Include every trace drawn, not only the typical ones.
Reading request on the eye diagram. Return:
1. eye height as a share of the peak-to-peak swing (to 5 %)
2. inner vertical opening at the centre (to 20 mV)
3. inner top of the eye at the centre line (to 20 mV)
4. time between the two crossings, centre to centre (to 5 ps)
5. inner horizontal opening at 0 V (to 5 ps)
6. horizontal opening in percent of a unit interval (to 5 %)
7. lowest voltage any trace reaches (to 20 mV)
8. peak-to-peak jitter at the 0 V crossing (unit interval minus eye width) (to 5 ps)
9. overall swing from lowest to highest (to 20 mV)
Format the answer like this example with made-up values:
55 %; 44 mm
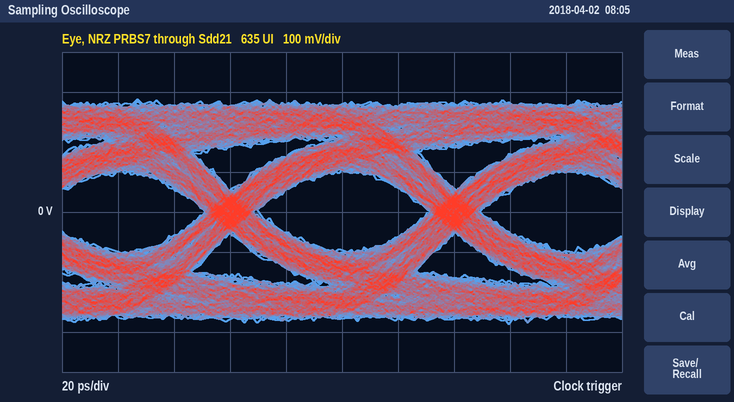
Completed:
35 %; 200 mV; 100 mV; 80 ps; 60 ps; 75 %; -280 mV; 20 ps; 560 mV
